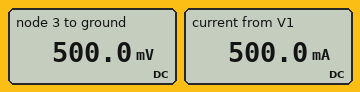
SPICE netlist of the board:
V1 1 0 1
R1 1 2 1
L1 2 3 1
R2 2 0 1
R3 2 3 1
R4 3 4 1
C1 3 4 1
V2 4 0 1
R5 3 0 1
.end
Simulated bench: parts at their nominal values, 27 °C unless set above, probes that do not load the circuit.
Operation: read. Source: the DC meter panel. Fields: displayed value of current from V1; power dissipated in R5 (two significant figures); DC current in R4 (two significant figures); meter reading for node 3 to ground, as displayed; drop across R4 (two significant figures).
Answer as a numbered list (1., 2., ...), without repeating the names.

1. 500.0 mA
2. 250 mW
3. 500 mA
4. 500.0 mV
5. 500 mV
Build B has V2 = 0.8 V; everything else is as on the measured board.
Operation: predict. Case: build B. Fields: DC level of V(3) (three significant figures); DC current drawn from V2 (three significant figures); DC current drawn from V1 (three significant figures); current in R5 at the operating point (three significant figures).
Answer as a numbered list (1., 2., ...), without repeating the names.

1. 450 mV
2. 350 mA
3. 550 mA
4. 450 mA
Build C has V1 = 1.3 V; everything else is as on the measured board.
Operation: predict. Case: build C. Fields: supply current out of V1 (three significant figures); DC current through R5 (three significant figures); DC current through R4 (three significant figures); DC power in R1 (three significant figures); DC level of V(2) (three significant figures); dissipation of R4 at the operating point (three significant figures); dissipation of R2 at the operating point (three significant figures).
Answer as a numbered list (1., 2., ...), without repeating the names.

1. 725 mA
2. 575 mA
3. 425 mA
4. 526 mW
5. 575 mV
6. 181 mW
7. 331 mW
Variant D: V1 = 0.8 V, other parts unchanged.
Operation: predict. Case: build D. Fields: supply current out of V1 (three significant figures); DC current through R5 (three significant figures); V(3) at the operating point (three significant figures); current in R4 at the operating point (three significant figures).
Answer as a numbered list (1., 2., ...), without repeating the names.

1. 350 mA
2. 450 mA
3. 450 mV
4. 550 mA
